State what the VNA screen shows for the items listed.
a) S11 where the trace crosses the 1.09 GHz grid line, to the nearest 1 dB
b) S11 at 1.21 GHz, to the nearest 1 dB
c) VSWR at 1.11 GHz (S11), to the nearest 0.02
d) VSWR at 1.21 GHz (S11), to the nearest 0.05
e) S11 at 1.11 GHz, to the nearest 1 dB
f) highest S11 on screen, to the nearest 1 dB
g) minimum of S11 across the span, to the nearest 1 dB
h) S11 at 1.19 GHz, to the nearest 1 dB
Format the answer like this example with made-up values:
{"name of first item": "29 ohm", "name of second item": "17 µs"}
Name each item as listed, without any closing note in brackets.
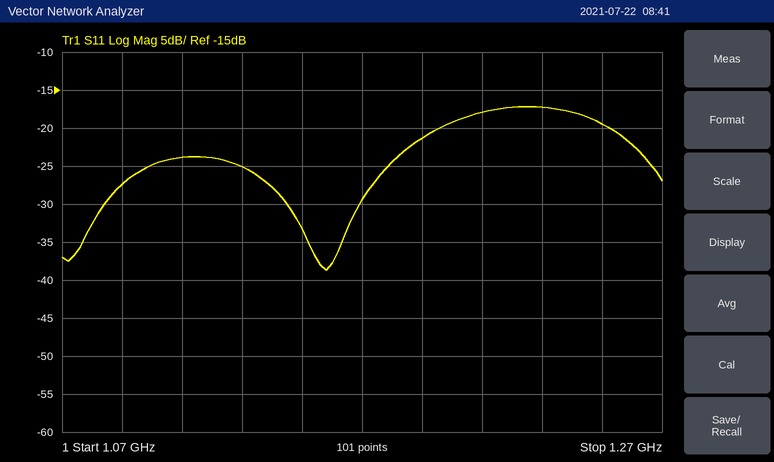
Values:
{"S11 where the trace crosses the 1.09 GHz grid line, to the nearest 1 dB": "-27 dB", "S11 at 1.21 GHz, to the nearest 1 dB": "-18 dB", "VSWR at 1.11 GHz (S11), to the nearest 0.02": "1.14", "VSWR at 1.21 GHz (S11), to the nearest 0.05": "1.30", "S11 at 1.11 GHz, to the nearest 1 dB": "-24 dB", "highest S11 on screen, to the nearest 1 dB": "-17 dB", "minimum of S11 across the span, to the nearest 1 dB": "-39 dB", "S11 at 1.19 GHz, to the nearest 1 dB": "-21 dB"}
